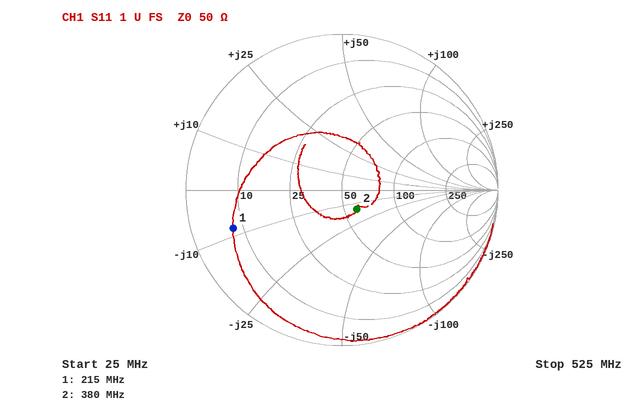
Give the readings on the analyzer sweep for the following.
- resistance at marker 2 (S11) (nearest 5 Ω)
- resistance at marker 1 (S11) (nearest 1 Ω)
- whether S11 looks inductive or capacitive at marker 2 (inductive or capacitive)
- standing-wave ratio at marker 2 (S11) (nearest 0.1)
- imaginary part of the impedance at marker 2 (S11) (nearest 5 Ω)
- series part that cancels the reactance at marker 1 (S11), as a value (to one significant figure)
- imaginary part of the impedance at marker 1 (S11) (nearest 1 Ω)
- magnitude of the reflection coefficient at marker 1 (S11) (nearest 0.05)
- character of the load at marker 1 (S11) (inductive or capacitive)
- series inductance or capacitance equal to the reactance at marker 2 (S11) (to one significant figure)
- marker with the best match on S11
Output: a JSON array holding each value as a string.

["60 Ω", "8 Ω", "capacitive", "1.4", "-15 Ω", "6 nH", "-8 Ω", "0.75", "capacitive", "30 pF", "marker 2"]
